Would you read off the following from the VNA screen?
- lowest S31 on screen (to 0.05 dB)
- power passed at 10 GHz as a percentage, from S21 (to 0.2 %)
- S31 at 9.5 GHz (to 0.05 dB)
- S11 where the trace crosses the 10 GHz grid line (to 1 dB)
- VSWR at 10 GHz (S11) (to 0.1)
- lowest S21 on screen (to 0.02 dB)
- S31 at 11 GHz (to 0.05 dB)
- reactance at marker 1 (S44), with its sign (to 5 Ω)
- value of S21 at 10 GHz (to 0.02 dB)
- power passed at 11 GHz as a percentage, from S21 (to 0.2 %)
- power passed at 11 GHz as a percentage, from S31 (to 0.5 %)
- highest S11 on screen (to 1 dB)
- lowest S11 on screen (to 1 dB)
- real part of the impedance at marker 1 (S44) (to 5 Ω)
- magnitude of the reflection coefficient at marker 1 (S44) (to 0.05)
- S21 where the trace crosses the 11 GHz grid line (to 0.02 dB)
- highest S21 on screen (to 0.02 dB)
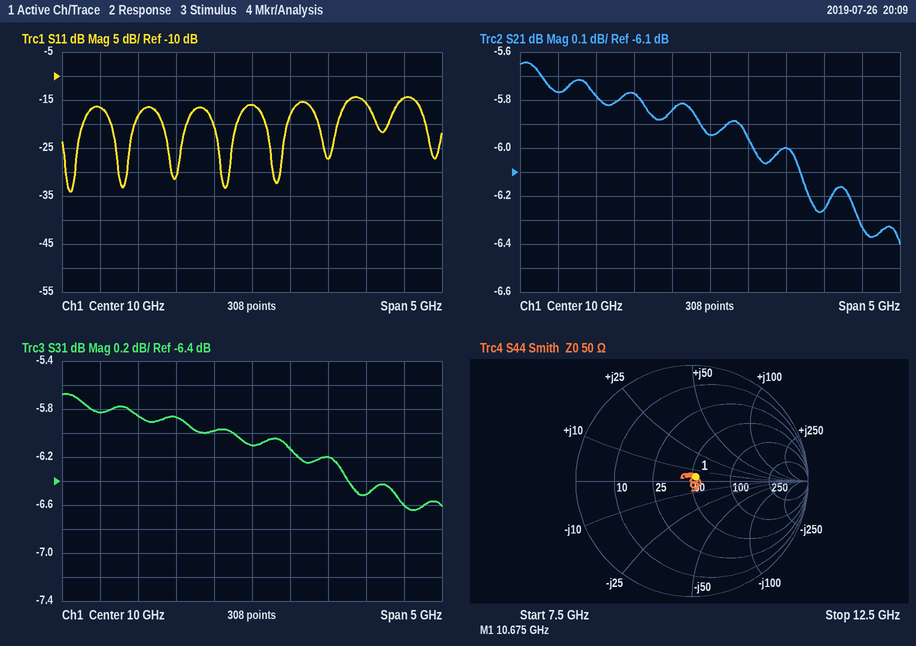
-6.65 dB
25.4 %
-6.00 dB
-16 dB
1.4
-6.40 dB
-6.20 dB
+5 Ω
-5.94 dB
25.2 %
24.0 %
-14 dB
-34 dB
55 Ω
0.05
-6.00 dB
-5.64 dB
